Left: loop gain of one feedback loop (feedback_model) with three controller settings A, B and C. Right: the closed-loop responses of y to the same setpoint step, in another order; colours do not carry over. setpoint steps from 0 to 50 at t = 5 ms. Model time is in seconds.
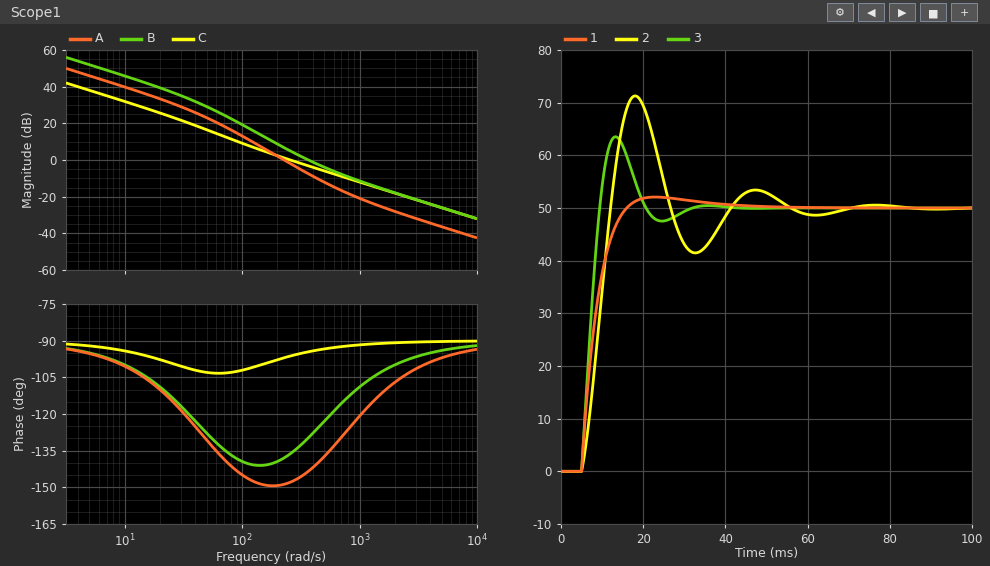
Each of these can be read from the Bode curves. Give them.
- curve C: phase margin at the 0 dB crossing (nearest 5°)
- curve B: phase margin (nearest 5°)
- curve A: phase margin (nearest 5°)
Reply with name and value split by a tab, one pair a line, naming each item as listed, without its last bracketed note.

curve C: phase margin at the 0 dB crossing	85°
curve B: phase margin	50°
curve A: phase margin	30°
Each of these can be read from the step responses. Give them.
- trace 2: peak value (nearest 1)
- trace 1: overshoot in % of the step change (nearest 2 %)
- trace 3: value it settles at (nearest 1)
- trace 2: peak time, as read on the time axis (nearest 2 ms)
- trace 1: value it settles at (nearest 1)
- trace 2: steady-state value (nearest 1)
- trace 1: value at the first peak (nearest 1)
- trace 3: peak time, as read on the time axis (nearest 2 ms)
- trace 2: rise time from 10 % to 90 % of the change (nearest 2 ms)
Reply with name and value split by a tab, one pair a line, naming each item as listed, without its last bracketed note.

trace 2: peak value	71
trace 1: overshoot in % of the step change	4 %
trace 3: value it settles at	50
trace 2: peak time, as read on the time axis	18 ms
trace 1: value it settles at	50
trace 2: steady-state value	50
trace 1: value at the first peak	52
trace 3: peak time, as read on the time axis	14 ms
trace 2: rise time from 10 % to 90 % of the change	6 ms
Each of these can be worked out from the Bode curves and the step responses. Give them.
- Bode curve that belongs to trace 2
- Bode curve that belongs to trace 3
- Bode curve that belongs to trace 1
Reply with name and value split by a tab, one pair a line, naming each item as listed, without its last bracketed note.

Bode curve that belongs to trace 2	A
Bode curve that belongs to trace 3	B
Bode curve that belongs to trace 1	C
